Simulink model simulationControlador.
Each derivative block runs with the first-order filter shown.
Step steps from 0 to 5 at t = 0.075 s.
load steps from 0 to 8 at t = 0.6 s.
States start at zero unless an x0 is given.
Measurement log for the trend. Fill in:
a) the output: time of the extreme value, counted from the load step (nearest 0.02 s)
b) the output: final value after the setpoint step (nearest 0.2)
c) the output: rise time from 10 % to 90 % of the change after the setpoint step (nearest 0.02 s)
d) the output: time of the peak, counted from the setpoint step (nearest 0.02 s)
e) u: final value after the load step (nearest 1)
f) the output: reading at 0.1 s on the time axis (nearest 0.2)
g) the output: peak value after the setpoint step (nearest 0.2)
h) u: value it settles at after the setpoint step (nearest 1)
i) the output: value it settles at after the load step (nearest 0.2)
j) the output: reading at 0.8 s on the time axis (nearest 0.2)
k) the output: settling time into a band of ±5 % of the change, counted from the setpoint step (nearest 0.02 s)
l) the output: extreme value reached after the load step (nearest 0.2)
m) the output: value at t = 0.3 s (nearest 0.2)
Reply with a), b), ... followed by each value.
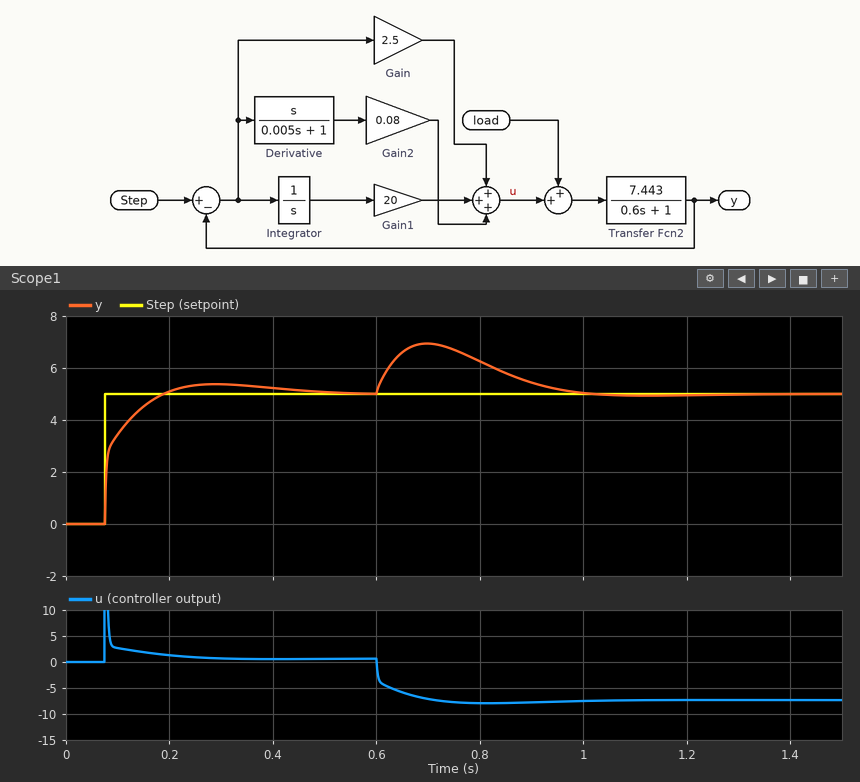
a) 0.10 s
b) 5.0
c) 0.08 s
d) 0.22 s
e) -7
f) 3.4
g) 5.4
h) 1
i) 5.0
j) 6.2
k) 0.32 s
l) 7.0
m) 5.4
